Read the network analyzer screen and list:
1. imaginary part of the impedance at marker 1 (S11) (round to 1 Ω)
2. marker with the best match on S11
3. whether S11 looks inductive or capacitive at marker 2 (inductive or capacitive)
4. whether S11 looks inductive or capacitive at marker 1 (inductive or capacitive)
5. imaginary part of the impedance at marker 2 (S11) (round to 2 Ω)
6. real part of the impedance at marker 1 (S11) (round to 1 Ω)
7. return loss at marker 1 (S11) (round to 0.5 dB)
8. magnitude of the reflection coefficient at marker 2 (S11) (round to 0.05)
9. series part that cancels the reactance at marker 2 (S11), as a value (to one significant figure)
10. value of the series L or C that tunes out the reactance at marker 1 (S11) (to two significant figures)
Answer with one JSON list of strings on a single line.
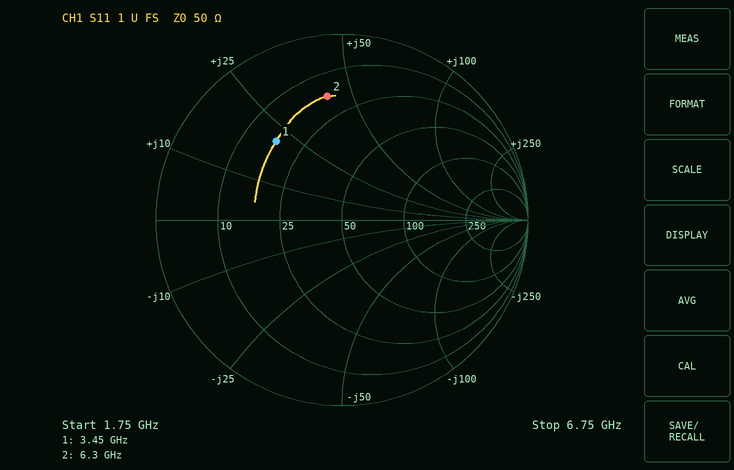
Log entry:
["+21 Ω", "marker 1", "inductive", "inductive", "+42 Ω", "17 Ω", "5.0 dB", "0.65", "600 fF", "2.2 pF"]
